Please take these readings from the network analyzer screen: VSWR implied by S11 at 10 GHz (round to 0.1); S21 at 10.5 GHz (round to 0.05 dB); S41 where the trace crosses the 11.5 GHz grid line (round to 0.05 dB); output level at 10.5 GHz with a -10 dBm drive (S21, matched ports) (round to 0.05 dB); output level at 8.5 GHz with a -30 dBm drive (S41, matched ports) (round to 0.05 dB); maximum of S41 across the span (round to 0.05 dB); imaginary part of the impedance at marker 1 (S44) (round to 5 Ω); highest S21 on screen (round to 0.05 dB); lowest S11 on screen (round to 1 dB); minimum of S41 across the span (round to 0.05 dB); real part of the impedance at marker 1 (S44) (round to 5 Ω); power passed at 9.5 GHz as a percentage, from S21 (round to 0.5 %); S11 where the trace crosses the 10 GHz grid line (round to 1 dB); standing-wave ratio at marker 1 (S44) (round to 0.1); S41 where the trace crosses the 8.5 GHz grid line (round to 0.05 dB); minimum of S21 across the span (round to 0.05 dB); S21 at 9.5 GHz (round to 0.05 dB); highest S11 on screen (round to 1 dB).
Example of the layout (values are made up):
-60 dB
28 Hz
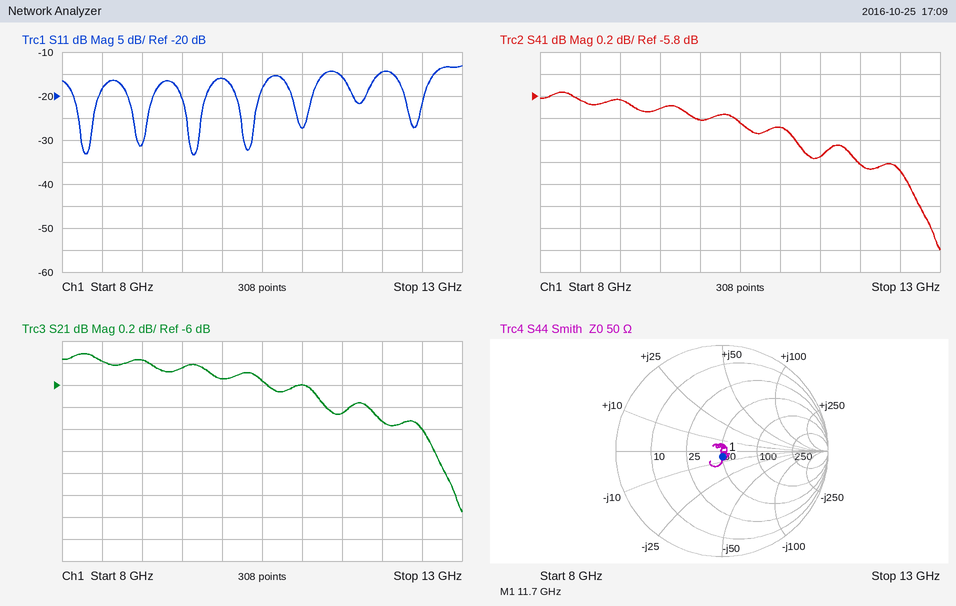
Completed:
1.4
-5.95 dB
-6.35 dB
-15.95 dBm
-35.85 dBm
-5.75 dB
-5 Ω
-5.70 dB
-33 dB
-7.20 dB
50 Ω
26.0 %
-16 dB
1.1
-5.85 dB
-7.15 dB
-5.85 dB
-13 dB
